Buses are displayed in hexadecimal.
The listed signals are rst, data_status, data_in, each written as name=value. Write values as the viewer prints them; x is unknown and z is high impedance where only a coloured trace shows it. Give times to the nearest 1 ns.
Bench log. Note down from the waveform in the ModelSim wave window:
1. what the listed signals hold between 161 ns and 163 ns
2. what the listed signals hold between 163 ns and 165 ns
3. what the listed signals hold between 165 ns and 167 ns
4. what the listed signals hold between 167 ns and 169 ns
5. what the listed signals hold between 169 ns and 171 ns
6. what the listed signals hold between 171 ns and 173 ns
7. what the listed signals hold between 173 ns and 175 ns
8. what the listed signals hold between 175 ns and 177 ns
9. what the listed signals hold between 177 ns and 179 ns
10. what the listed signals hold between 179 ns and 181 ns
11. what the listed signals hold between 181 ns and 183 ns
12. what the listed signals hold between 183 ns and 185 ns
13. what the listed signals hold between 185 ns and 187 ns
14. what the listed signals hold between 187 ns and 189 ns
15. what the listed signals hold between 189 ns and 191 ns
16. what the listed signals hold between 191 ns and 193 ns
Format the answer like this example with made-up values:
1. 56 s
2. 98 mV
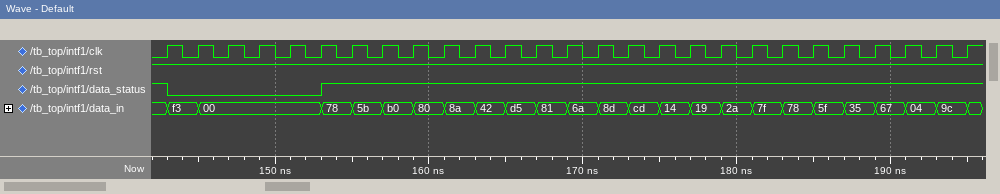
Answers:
1. rst=1, data_status=1, data_in=8a
2. rst=1, data_status=1, data_in=42
3. rst=1, data_status=1, data_in=d5
4. rst=1, data_status=1, data_in=81
5. rst=1, data_status=1, data_in=6a
6. rst=1, data_status=1, data_in=8d
7. rst=1, data_status=1, data_in=cd
8. rst=1, data_status=1, data_in=14
9. rst=1, data_status=1, data_in=19
10. rst=1, data_status=1, data_in=2a
11. rst=1, data_status=1, data_in=7f
12. rst=1, data_status=1, data_in=78
13. rst=1, data_status=1, data_in=5f
14. rst=1, data_status=1, data_in=35
15. rst=1, data_status=1, data_in=67
16. rst=1, data_status=1, data_in=04
